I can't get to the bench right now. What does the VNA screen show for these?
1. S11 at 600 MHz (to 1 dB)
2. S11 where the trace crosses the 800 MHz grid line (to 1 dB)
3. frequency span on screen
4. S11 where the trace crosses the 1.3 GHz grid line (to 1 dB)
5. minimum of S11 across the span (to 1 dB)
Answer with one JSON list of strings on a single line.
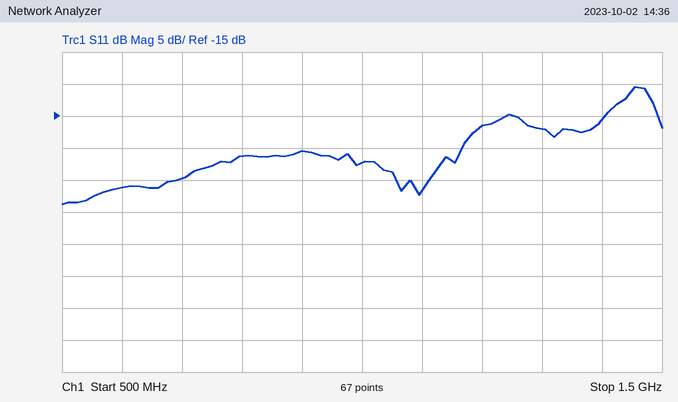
["-26 dB", "-21 dB", "1 GHz", "-17 dB", "-29 dB"]
